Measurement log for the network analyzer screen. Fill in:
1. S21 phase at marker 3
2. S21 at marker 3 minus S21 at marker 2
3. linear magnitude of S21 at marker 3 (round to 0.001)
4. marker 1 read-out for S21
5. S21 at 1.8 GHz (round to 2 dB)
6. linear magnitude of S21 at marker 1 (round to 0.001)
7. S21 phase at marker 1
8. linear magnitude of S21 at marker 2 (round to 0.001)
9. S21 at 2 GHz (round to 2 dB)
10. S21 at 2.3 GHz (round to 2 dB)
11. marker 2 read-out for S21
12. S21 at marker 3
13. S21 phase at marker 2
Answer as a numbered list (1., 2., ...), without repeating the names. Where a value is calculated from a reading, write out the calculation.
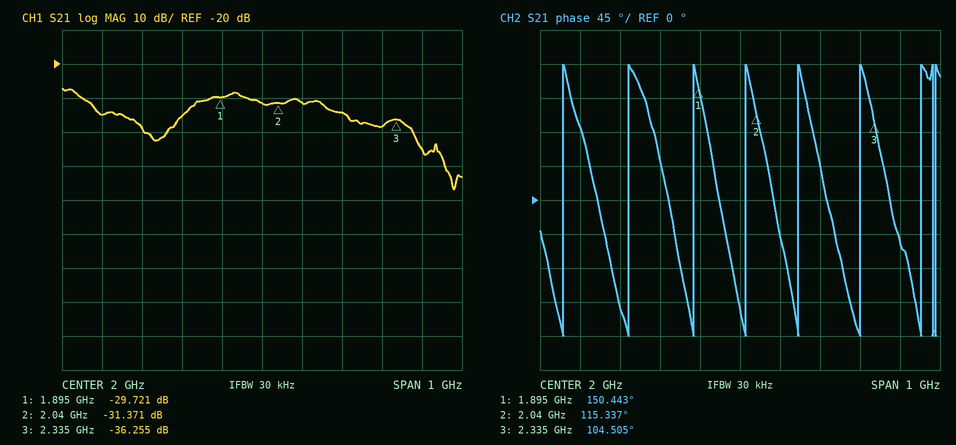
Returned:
1. 104.505°
2. -36.255 − (-31.371) = -4.884 dB
3. 10^(-36.255/20) ≈ 0.015
4. -29.721 dB
5. -36 dB
6. 10^(-29.721/20) ≈ 0.033
7. 150.443°
8. 10^(-31.371/20) ≈ 0.027
9. -32 dB
10. -38 dB
11. -31.371 dB
12. -36.255 dB
13. 115.337°
